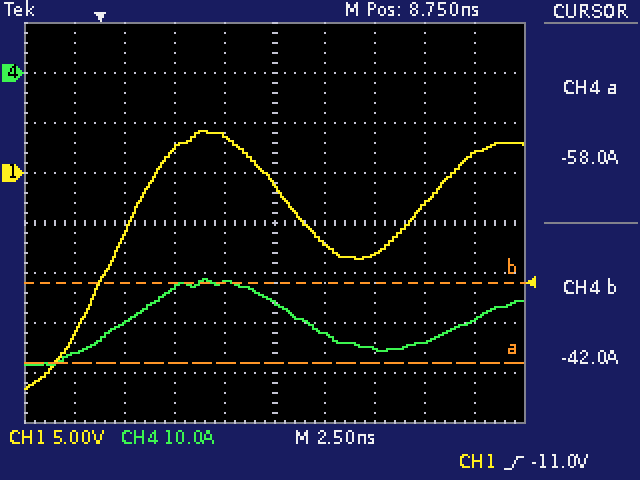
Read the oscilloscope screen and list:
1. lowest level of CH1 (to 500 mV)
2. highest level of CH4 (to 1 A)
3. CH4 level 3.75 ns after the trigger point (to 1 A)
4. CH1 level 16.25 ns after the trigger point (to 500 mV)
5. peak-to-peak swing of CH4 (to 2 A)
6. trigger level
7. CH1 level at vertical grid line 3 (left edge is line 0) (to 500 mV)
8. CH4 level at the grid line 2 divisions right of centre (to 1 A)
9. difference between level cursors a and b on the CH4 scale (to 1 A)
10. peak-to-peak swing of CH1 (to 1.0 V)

-21.5 V
-41 A
-43 A
-3.0 V
18 A
-11.0 V
2.5 V
-55 A
16 A
26.0 V
